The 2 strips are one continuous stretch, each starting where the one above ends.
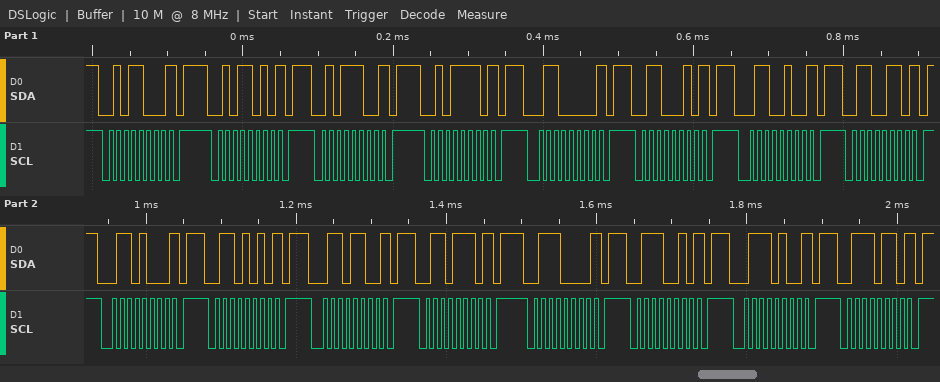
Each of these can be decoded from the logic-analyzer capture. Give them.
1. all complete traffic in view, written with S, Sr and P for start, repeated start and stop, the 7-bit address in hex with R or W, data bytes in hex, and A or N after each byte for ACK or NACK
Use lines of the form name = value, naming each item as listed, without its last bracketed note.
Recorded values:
all complete traffic in view, written with S, Sr and P for start, repeated start and stop, the 7-bit address in hex with R or W, data bytes in hex, and A or N after each byte for ACK or NACK = S 2CW N P S 2DW N P S 2EW N P S 2FW N P S 30W N P S 31W N P S 32W N P S 33W N P S 34W N P S 35W N P S 36W N P S 37W N P S 38W N P S 39W N P S 3AW N P S 3BW N P
